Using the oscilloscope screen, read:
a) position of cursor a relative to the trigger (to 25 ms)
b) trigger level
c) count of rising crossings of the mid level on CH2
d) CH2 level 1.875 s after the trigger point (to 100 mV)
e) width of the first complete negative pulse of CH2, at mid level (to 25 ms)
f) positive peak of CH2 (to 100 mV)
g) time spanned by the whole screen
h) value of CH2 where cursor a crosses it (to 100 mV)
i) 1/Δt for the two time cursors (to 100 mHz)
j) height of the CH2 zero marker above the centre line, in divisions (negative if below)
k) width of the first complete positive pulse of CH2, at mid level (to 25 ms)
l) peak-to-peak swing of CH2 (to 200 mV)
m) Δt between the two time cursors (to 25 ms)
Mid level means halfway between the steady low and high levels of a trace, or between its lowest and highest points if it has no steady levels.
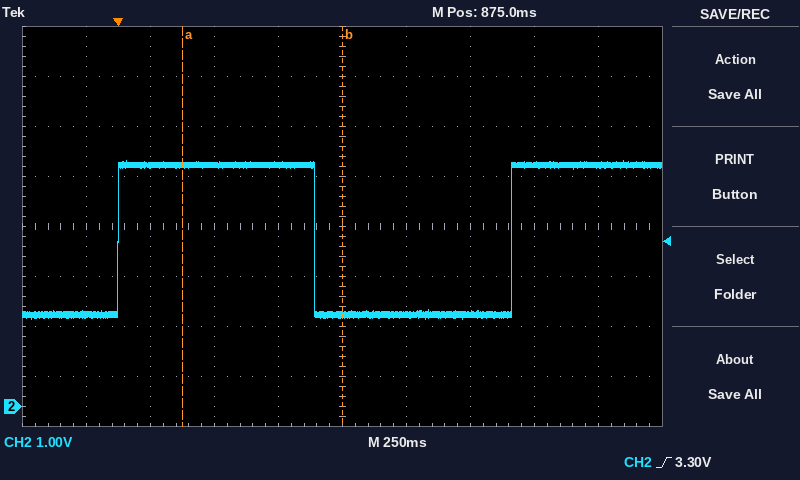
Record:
+250 ms
3.30 V
2
4.8 V
775 ms
4.9 V
2.5 s
4.8 V
1.6 Hz
-3.6 div
775 ms
3.2 V
625 ms
